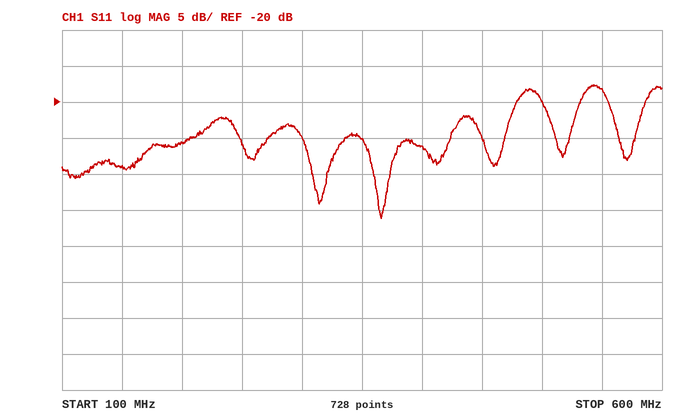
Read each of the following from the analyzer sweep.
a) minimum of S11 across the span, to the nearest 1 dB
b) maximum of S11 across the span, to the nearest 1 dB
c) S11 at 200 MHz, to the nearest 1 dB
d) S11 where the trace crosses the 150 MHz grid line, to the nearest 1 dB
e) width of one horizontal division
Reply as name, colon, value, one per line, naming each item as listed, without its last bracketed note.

minimum of S11 across the span, to the nearest 1 dB: -36 dB
maximum of S11 across the span, to the nearest 1 dB: -18 dB
S11 at 200 MHz, to the nearest 1 dB: -26 dB
S11 where the trace crosses the 150 MHz grid line, to the nearest 1 dB: -29 dB
width of one horizontal division: 50 MHz
